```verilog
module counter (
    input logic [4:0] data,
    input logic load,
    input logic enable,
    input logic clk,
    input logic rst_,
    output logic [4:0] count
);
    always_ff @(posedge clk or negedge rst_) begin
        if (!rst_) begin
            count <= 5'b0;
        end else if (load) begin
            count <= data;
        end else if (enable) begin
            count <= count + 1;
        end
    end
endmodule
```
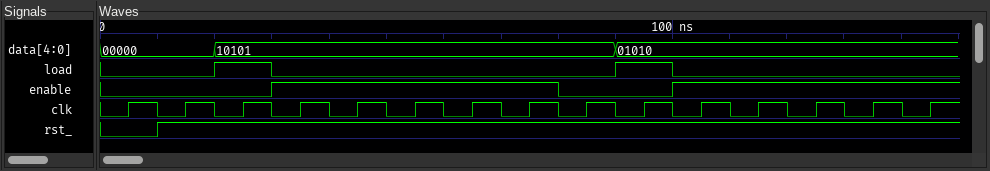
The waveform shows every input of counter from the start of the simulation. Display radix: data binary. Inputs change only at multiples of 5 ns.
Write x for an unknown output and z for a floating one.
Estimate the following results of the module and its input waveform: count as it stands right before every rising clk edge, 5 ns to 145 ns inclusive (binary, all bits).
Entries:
00000, 00000, 00000, 10101, 10110, 10111, 11000, 11001, 11010, 11010, 01010, 01011, 01100, 01101, 01110
